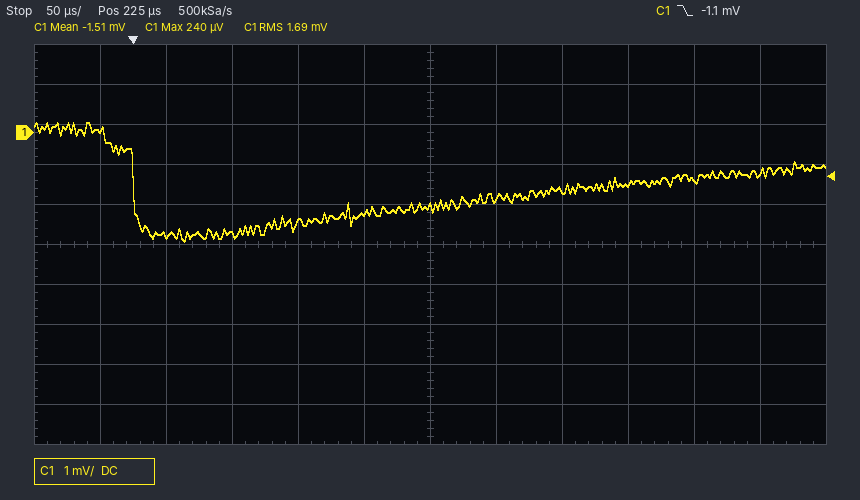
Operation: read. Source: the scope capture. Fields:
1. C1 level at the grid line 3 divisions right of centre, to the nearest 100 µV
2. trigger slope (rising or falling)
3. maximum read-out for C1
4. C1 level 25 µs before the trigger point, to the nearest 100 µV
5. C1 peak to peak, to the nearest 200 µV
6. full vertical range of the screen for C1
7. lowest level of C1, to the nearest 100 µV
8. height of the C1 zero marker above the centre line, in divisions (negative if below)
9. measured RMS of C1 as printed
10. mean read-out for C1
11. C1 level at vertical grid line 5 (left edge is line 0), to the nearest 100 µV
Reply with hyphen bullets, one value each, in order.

- -1.3 mV
- falling
- 240 µV
- 100 µV
- 3.0 mV
- 10 mV
- -2.7 mV
- +2.8 div
- 1.69 mV
- -1.51 mV
- -2.0 mV
